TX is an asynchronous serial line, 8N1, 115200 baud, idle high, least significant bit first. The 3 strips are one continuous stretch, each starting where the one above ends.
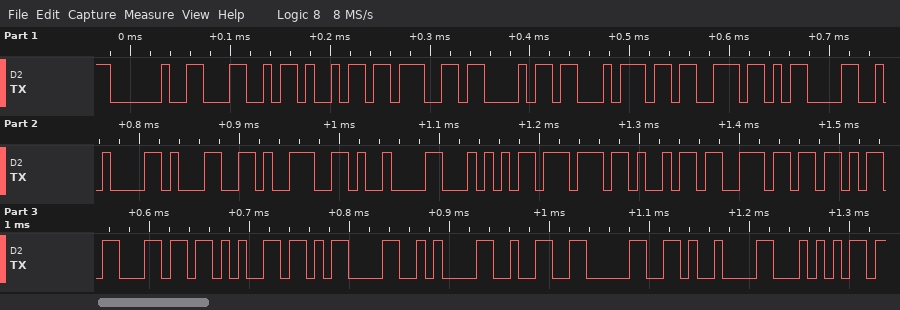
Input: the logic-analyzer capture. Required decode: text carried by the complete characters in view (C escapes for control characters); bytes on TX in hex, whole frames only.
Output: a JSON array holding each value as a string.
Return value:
["\" Lights\\r\\n19\\tTwinkle\\r\\n20\\tT\"", "20 4C 69 67 68 74 73 0D 0A 31 39 09 54 77 69 6E 6B 6C 65 0D 0A 32 30 09 54"]
